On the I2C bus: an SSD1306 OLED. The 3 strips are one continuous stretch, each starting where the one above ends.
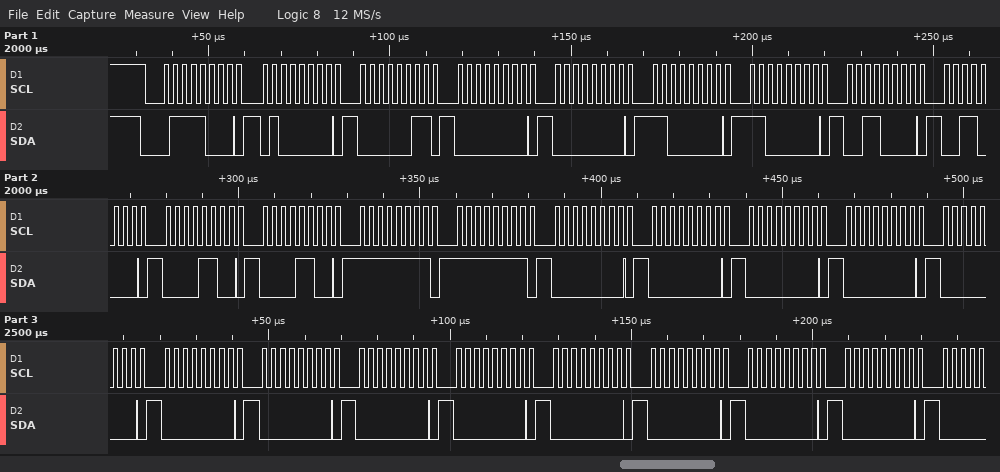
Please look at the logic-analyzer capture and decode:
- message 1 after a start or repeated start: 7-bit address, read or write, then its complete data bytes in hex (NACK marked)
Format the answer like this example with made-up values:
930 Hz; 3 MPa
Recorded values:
0x3C write: 40 03 00 00 C0 C0 30 30 0C 0C FF FF 00 00 00 00 00 00 00 00 00 00 00 00 00
